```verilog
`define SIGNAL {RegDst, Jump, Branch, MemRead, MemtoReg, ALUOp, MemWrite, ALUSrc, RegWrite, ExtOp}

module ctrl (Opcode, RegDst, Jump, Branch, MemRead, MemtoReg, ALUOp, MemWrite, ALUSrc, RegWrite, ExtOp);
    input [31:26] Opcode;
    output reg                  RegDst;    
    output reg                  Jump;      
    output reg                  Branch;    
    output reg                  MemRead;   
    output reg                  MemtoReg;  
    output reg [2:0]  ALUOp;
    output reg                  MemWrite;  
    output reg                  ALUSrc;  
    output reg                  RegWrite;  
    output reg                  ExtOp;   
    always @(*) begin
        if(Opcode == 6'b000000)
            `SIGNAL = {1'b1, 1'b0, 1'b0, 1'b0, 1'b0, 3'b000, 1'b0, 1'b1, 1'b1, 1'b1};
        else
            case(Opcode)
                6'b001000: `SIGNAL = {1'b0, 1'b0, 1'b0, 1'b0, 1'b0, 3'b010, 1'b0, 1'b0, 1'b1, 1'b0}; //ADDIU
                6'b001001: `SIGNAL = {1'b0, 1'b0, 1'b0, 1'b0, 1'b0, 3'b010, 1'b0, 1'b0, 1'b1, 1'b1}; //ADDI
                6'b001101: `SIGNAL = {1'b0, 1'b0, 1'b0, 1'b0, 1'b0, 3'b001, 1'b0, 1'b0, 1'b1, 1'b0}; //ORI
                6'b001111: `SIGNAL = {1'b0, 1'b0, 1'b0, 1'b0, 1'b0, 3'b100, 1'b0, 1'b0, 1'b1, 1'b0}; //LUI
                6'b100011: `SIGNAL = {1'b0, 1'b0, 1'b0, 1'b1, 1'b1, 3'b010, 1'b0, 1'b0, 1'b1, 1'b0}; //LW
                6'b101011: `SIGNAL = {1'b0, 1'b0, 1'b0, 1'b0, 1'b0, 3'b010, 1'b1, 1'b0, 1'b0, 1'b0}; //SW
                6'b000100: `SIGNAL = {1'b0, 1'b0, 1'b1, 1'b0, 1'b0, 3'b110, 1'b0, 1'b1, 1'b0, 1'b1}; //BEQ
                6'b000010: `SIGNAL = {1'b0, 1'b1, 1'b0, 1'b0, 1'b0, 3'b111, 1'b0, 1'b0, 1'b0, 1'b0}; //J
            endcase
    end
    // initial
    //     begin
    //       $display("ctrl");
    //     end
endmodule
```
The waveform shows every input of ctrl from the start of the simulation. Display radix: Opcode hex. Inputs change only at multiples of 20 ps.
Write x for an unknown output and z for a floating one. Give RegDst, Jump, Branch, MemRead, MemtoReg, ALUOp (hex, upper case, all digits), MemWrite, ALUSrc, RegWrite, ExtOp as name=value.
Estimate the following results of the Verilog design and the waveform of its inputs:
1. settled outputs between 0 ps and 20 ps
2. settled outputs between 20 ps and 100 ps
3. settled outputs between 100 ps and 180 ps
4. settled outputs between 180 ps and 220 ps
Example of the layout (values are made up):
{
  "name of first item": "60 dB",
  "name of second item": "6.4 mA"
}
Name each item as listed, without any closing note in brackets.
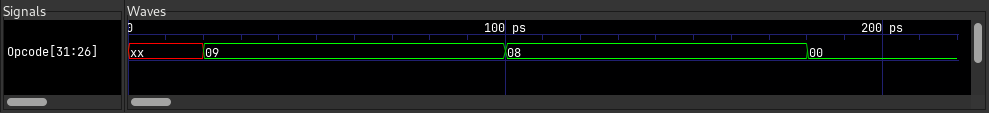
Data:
{
  "settled outputs between 0 ps and 20 ps": "RegDst=x, Jump=x, Branch=x, MemRead=x, MemtoReg=x, ALUOp=x, MemWrite=x, ALUSrc=x, RegWrite=x, ExtOp=x",
  "settled outputs between 20 ps and 100 ps": "RegDst=0, Jump=0, Branch=0, MemRead=0, MemtoReg=0, ALUOp=2, MemWrite=0, ALUSrc=0, RegWrite=1, ExtOp=1",
  "settled outputs between 100 ps and 180 ps": "RegDst=0, Jump=0, Branch=0, MemRead=0, MemtoReg=0, ALUOp=2, MemWrite=0, ALUSrc=0, RegWrite=1, ExtOp=0",
  "settled outputs between 180 ps and 220 ps": "RegDst=1, Jump=0, Branch=0, MemRead=0, MemtoReg=0, ALUOp=0, MemWrite=0, ALUSrc=1, RegWrite=1, ExtOp=1"
}
